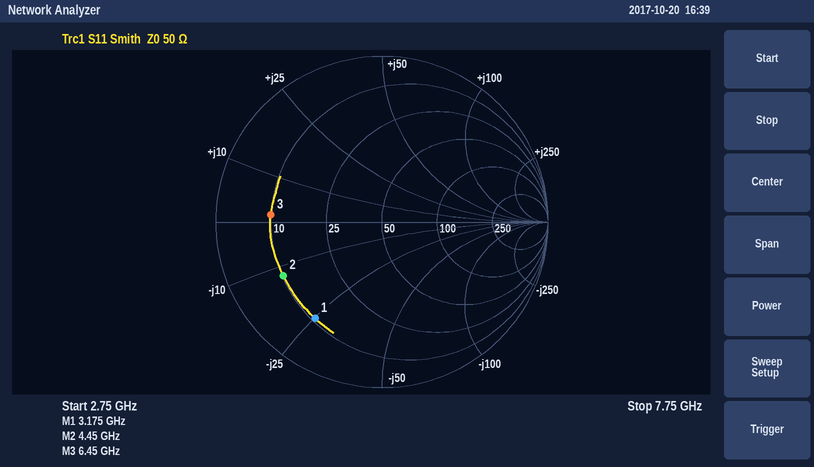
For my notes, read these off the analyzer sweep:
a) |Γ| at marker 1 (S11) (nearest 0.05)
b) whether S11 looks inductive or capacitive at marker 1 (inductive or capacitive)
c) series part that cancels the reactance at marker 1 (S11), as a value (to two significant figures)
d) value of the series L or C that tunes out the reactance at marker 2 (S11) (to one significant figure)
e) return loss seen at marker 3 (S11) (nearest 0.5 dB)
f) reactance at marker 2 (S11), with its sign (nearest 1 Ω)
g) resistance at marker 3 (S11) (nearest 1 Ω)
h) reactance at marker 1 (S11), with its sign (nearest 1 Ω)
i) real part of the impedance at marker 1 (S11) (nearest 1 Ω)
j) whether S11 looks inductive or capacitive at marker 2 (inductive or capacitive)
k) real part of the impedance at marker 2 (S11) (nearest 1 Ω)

0.70
capacitive
1.3 nH
400 pH
3.5 dB
-12 Ω
10 Ω
-25 Ω
11 Ω
capacitive
10 Ω
